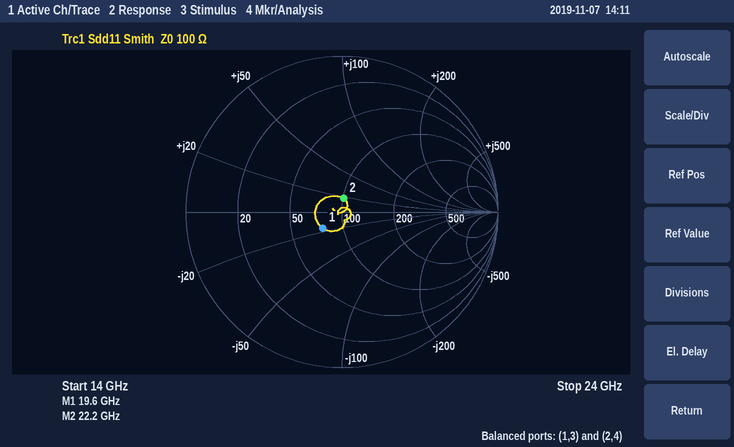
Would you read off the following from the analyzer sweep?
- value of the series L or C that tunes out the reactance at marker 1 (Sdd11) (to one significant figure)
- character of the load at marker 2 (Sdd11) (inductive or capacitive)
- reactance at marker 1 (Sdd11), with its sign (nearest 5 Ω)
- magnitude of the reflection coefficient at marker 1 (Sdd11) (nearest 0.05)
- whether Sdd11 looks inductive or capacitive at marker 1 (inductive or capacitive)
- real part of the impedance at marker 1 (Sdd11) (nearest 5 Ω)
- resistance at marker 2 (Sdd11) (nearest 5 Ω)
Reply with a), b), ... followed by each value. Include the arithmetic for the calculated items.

a) L = 15 Ω/(2π × 19.6 GHz) ≈ 122 pH, so 100 pH to one significant figure
b) inductive
c) -15 Ω
d) 0.15
e) capacitive
f) 75 Ω
g) 100 Ω
